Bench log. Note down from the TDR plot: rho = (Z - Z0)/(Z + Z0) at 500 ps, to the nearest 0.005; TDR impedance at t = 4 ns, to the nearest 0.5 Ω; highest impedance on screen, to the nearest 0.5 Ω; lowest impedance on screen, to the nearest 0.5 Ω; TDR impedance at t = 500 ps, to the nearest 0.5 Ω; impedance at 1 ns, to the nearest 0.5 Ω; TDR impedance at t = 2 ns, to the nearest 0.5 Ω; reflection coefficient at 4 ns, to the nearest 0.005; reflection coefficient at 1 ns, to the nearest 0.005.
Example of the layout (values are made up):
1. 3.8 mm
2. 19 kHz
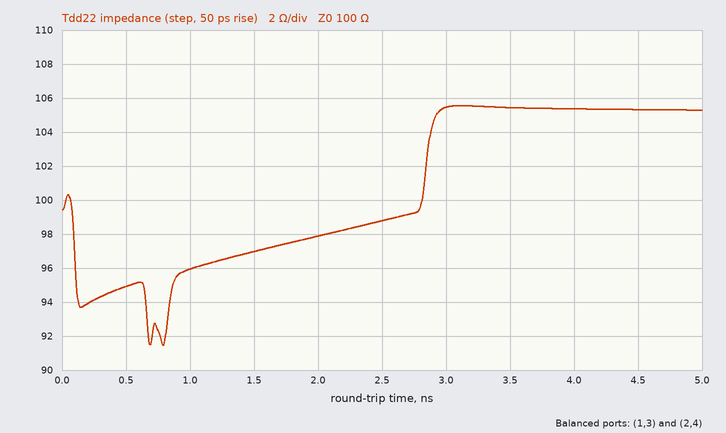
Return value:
1. -0.025
2. 105.5 Ω
3. 105.5 Ω
4. 91.5 Ω
5. 95.0 Ω
6. 96.0 Ω
7. 98.0 Ω
8. +0.025
9. -0.020
